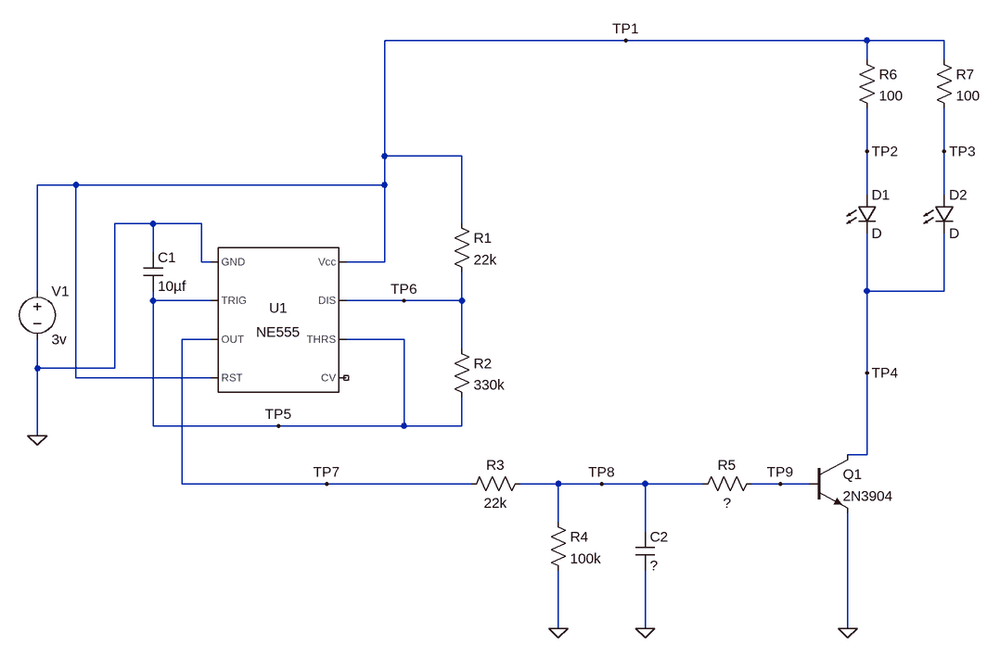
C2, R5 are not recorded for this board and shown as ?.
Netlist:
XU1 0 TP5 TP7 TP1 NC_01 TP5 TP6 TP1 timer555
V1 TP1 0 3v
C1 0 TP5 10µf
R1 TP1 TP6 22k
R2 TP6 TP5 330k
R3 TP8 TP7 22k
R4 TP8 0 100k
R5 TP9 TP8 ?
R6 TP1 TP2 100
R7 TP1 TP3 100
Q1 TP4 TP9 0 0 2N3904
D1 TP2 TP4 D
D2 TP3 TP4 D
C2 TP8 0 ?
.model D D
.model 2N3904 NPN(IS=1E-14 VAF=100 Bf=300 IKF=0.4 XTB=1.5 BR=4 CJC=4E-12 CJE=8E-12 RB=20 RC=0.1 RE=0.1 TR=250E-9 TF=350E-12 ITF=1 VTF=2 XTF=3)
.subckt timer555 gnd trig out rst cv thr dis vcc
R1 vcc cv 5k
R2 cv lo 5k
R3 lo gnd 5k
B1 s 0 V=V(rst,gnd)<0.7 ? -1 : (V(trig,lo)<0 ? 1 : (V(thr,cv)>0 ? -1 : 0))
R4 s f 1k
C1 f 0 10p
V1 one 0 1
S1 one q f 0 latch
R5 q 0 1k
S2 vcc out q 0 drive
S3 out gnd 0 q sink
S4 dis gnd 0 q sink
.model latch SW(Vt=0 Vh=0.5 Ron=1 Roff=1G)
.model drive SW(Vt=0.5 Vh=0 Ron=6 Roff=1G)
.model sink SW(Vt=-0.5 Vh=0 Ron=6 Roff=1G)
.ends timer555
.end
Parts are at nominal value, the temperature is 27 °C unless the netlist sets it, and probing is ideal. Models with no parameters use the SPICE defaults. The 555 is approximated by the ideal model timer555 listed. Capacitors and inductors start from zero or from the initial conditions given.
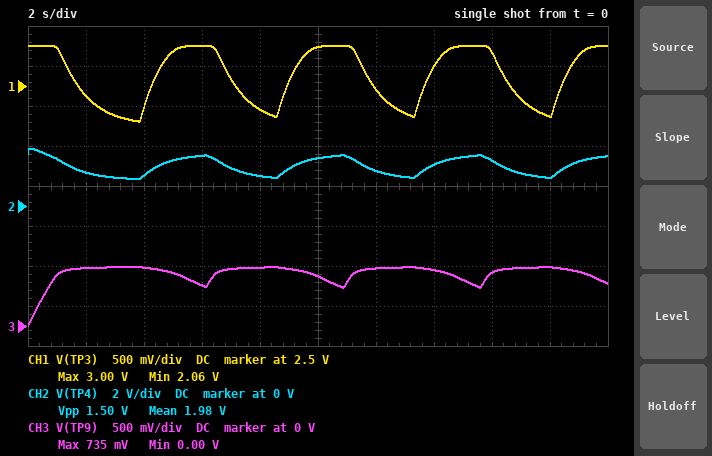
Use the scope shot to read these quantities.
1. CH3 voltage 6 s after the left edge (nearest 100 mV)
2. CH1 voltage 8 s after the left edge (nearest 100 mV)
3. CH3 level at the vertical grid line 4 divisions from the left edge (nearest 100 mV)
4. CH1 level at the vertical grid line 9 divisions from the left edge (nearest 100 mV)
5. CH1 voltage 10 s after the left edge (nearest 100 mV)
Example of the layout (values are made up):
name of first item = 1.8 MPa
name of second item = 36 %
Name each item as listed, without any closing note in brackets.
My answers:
CH3 voltage 6 s after the left edge = 500 mV
CH1 voltage 8 s after the left edge = 2.2 V
CH3 level at the vertical grid line 4 divisions from the left edge = 700 mV
CH1 level at the vertical grid line 9 divisions from the left edge = 2.1 V
CH1 voltage 10 s after the left edge = 3.0 V
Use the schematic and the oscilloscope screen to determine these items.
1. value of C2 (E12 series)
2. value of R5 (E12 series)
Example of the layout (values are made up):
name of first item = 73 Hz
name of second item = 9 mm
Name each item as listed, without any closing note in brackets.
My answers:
value of C2 = 180 µF
value of R5 = 6.8 kΩ
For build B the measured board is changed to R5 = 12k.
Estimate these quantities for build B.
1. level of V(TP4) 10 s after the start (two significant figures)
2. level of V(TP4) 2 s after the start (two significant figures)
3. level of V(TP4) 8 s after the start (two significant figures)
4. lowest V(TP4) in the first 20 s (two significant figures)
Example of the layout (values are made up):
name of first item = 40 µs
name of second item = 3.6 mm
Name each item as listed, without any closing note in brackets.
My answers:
level of V(TP4) 10 s after the start = 2.3 V
level of V(TP4) 2 s after the start = 1.9 V
level of V(TP4) 8 s after the start = 1.7 V
lowest V(TP4) in the first 20 s = 1.6 V
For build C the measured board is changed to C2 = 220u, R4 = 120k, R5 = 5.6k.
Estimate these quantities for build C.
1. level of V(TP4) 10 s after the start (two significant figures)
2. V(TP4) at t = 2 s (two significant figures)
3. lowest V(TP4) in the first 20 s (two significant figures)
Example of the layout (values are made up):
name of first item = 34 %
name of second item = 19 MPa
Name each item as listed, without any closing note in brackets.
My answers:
level of V(TP4) 10 s after the start = 2.3 V
V(TP4) at t = 2 s = 1.8 V
lowest V(TP4) in the first 20 s = 1.3 V
